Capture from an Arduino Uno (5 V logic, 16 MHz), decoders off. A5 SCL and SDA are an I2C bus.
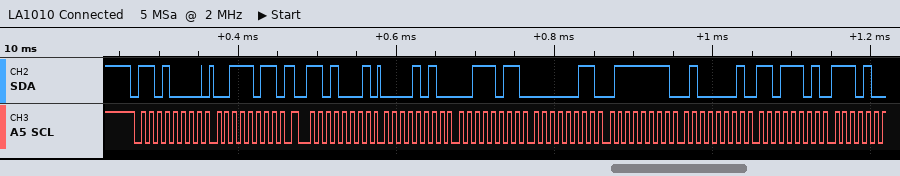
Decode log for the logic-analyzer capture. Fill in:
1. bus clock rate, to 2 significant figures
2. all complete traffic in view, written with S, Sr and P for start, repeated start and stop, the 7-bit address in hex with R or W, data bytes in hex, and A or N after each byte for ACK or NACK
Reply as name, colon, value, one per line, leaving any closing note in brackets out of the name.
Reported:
bus clock rate, to 2 significant figures: 100 kHz
all complete traffic in view, written with S, Sr and P for start, repeated start and stop, the 7-bit address in hex with R or W, data bytes in hex, and A or N after each byte for ACK or NACK: S 68W A 3B A Sr 68R A 0A A 3B A 03 A 7F A 41 A DD A
